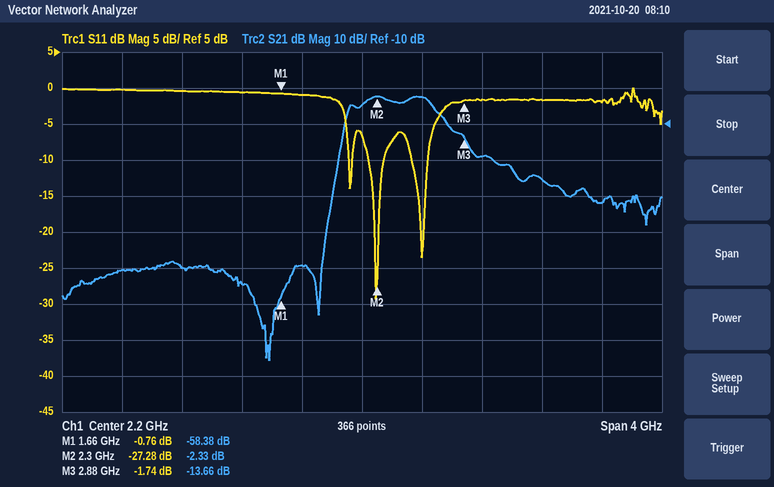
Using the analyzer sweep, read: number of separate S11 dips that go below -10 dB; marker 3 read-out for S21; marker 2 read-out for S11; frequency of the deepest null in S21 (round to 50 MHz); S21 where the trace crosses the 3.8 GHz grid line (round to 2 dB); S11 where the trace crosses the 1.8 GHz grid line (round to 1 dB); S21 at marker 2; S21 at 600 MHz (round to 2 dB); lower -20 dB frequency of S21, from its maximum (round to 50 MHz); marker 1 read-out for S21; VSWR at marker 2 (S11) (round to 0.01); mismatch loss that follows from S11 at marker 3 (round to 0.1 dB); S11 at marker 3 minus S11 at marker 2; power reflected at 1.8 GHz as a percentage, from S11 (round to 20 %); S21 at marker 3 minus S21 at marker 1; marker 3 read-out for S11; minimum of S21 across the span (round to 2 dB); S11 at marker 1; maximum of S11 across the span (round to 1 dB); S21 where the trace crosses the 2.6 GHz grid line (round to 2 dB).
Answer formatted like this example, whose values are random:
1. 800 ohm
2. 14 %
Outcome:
1. 3
2. -13.66 dB
3. -27.28 dB
4. 1.60 GHz
5. -32 dB
6. -1 dB
7. -2.33 dB
8. -50 dB
9. 2.05 GHz
10. -58.38 dB
11. 1.09
12. 4.8 dB
13. 25.54 dB
14. 80 %
15. 44.72 dB
16. -1.74 dB
17. -76 dB
18. -0.76 dB
19. 0 dB
20. -2 dB
